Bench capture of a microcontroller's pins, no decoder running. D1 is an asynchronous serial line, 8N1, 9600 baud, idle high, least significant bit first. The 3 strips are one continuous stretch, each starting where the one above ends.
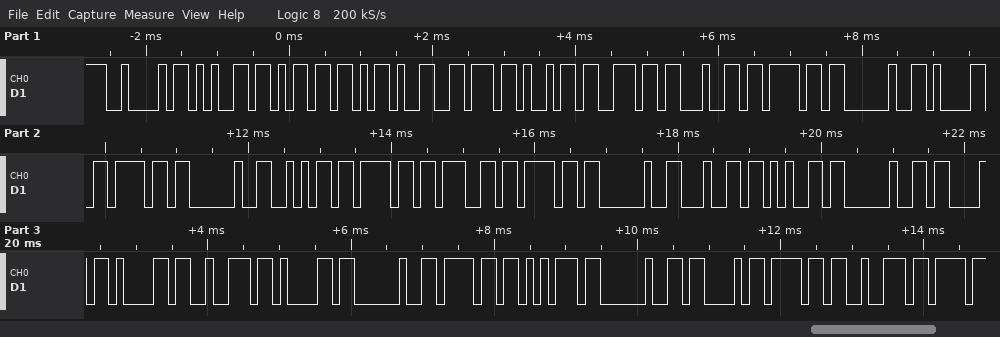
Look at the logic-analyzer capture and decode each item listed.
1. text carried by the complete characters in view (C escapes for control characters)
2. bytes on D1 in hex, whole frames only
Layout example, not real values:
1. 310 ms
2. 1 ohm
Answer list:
1. "Bem-vindo ao jogo de Cara ou Cor"
2. 42 65 6D 2D 76 69 6E 64 6F 20 61 6F 20 6A 6F 67 6F 20 64 65 20 43 61 72 61 20 6F 75 20 43 6F 72
